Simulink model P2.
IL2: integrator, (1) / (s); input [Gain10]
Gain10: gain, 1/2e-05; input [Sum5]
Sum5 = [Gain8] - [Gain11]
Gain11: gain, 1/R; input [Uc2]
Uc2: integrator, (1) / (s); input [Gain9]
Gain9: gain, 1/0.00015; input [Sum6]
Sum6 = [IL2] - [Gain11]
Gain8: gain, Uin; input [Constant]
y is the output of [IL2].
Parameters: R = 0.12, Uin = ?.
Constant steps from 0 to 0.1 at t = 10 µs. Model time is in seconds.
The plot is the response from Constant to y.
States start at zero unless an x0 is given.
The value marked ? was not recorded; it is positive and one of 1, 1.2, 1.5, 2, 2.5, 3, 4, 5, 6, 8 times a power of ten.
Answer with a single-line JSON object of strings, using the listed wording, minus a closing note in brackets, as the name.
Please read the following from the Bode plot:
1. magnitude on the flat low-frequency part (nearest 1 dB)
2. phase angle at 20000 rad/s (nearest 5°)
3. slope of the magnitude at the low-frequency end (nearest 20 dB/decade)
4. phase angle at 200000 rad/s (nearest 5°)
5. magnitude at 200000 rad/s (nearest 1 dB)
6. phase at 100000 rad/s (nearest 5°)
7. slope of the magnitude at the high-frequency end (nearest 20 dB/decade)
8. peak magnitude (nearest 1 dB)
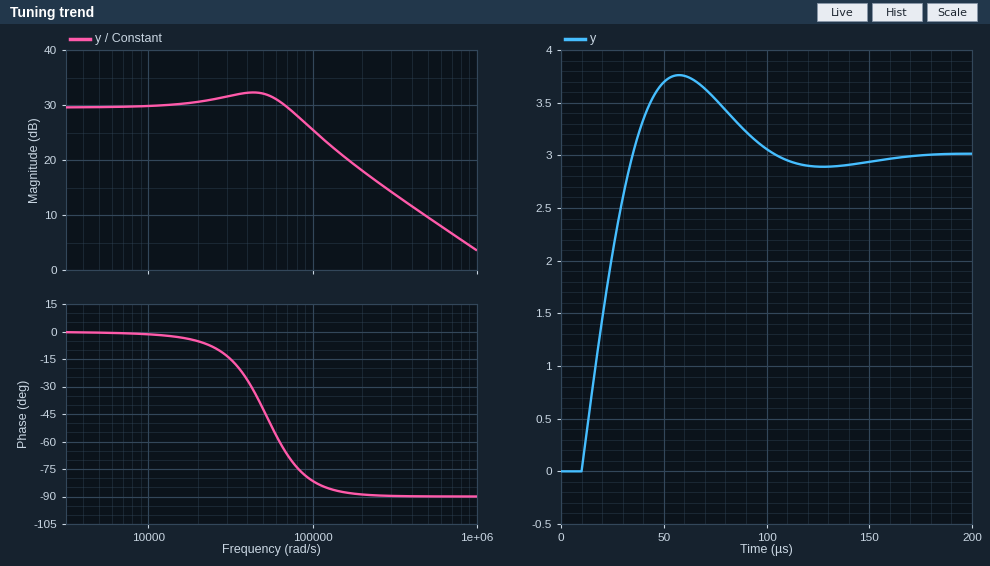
{"magnitude on the flat low-frequency part": "30 dB", "phase angle at 20000 rad/s": "-5°", "slope of the magnitude at the low-frequency end": "0 dB/decade", "phase angle at 200000 rad/s": "-90°", "magnitude at 200000 rad/s": "18 dB", "phase at 100000 rad/s": "-80°", "slope of the magnitude at the high-frequency end": "-20 dB/decade", "peak magnitude": "32 dB"}
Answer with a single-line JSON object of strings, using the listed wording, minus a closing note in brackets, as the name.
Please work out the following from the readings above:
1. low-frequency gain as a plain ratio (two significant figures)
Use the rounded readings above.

{"low-frequency gain as a plain ratio": "32"}
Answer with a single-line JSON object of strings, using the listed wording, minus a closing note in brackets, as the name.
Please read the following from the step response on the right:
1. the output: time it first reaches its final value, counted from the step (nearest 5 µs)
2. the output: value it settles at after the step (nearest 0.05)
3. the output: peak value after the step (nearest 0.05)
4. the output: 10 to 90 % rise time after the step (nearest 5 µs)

{"the output: time it first reaches its final value, counted from the step": "25 µs", "the output: value it settles at after the step": "3.00", "the output: peak value after the step": "3.75", "the output: 10 to 90 % rise time after the step": "20 µs"}
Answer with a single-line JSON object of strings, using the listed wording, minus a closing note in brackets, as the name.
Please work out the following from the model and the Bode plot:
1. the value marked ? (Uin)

{"the value marked ?": "30"}
